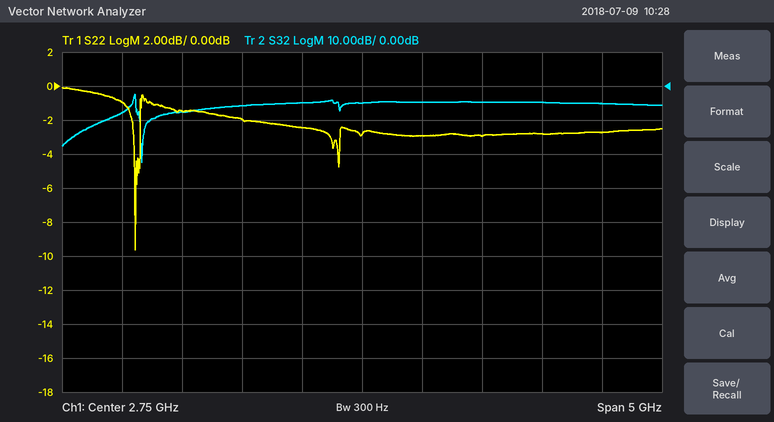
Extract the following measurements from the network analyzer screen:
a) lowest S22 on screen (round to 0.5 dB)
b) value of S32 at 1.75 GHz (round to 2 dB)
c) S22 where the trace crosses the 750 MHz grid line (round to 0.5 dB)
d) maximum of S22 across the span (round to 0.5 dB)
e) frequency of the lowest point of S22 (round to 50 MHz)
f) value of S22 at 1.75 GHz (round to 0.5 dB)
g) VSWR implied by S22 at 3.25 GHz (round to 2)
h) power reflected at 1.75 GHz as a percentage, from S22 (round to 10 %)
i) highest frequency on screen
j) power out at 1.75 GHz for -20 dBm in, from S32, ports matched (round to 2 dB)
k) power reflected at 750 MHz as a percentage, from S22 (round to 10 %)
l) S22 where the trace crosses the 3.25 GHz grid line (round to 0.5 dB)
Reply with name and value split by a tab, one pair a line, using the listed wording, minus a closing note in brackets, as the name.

lowest S22 on screen	-9.5 dB
value of S32 at 1.75 GHz	-6 dB
S22 where the trace crosses the 750 MHz grid line	-1.0 dB
maximum of S22 across the span	0.0 dB
frequency of the lowest point of S22	850 MHz
value of S22 at 1.75 GHz	-2.0 dB
VSWR implied by S22 at 3.25 GHz	6
power reflected at 1.75 GHz as a percentage, from S22	60 %
highest frequency on screen	5.25 GHz
power out at 1.75 GHz for -20 dBm in, from S32, ports matched	-26 dBm
power reflected at 750 MHz as a percentage, from S22	80 %
S22 where the trace crosses the 3.25 GHz grid line	-3.0 dB
